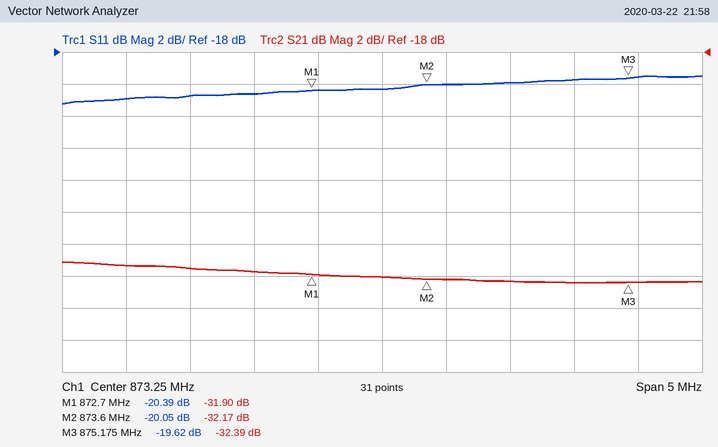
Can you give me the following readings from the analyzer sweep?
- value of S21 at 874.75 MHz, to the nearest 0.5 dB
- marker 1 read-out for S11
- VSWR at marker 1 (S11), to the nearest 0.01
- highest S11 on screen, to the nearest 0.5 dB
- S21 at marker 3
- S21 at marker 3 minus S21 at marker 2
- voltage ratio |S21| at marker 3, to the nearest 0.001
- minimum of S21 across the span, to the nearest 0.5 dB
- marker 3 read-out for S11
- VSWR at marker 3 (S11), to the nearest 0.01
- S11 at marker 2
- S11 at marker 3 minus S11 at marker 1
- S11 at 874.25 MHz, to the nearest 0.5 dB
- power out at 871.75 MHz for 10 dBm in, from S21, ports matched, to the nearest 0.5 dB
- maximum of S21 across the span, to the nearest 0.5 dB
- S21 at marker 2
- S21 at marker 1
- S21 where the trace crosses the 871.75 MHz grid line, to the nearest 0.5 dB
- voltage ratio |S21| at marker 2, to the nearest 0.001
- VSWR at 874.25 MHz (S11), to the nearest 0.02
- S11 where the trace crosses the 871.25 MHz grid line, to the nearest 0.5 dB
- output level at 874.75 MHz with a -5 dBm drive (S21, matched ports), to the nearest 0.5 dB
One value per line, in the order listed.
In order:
-32.5 dB
-20.39 dB
1.21
-19.5 dB
-32.39 dB
-0.22 dB
0.024
-32.5 dB
-19.62 dB
1.23
-20.05 dB
0.77 dB
-20.0 dB
-21.5 dBm
-31.0 dB
-32.17 dB
-31.90 dB
-31.5 dB
0.025
1.22
-21.0 dB
-37.5 dBm
